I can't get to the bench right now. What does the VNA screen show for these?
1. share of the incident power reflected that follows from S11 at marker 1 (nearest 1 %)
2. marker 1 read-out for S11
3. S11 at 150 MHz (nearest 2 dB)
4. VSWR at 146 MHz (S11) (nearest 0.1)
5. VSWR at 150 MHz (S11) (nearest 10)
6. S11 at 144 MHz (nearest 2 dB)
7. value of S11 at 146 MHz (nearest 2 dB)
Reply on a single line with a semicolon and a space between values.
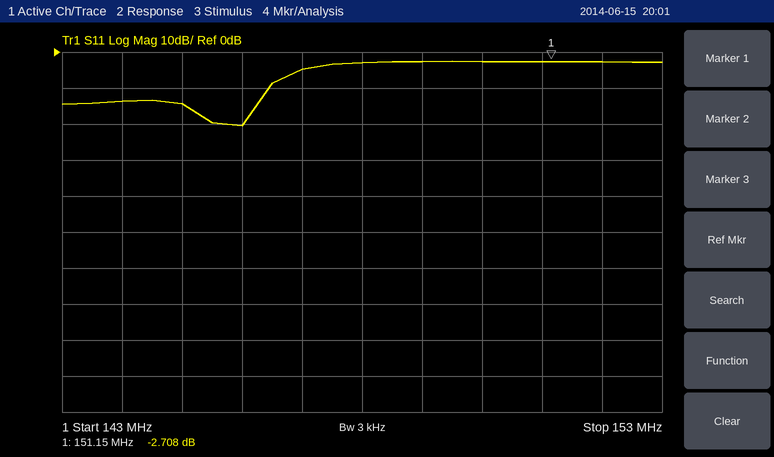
54 %; -2.708 dB; -2 dB; 1.2; 10; -14 dB; -20 dB
